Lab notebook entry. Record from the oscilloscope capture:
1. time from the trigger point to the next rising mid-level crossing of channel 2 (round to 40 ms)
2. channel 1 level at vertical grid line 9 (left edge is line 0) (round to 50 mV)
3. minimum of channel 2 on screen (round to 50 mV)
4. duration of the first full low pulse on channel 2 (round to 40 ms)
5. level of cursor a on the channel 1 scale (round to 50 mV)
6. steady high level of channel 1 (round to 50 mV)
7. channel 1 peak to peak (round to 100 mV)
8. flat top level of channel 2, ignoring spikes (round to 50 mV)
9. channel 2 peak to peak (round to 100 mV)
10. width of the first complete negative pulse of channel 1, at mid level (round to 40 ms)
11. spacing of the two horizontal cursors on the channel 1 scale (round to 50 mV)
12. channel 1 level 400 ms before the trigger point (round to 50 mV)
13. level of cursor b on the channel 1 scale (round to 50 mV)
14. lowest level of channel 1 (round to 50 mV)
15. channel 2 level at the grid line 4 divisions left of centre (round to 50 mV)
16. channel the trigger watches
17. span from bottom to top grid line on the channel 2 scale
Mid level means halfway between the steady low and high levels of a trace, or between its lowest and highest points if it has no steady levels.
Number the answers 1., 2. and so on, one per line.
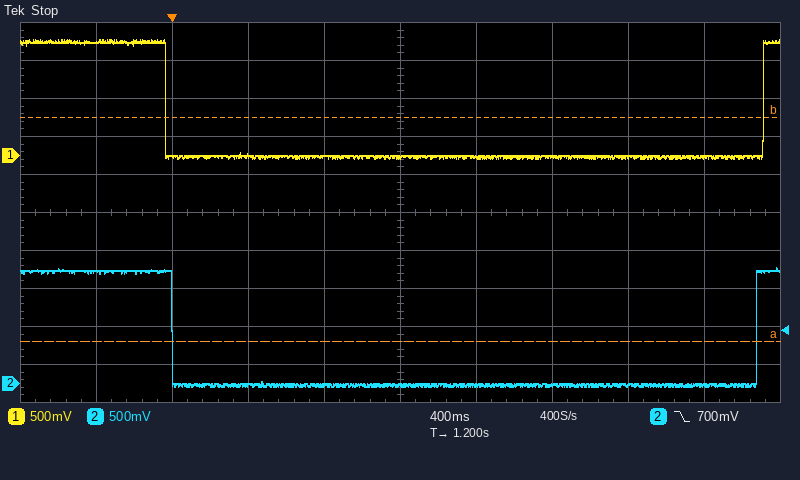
1. 3.08 s
2. 0 mV
3. -50 mV
4. 3.08 s
5. -2.45 V
6. 1.50 V
7. 1.60 V
8. 1.50 V
9. 1.60 V
10. 3.16 s
11. 2.95 V
12. 1.50 V
13. 500 mV
14. -50 mV
15. 1.45 V
16. channel 2
17. 5 V
